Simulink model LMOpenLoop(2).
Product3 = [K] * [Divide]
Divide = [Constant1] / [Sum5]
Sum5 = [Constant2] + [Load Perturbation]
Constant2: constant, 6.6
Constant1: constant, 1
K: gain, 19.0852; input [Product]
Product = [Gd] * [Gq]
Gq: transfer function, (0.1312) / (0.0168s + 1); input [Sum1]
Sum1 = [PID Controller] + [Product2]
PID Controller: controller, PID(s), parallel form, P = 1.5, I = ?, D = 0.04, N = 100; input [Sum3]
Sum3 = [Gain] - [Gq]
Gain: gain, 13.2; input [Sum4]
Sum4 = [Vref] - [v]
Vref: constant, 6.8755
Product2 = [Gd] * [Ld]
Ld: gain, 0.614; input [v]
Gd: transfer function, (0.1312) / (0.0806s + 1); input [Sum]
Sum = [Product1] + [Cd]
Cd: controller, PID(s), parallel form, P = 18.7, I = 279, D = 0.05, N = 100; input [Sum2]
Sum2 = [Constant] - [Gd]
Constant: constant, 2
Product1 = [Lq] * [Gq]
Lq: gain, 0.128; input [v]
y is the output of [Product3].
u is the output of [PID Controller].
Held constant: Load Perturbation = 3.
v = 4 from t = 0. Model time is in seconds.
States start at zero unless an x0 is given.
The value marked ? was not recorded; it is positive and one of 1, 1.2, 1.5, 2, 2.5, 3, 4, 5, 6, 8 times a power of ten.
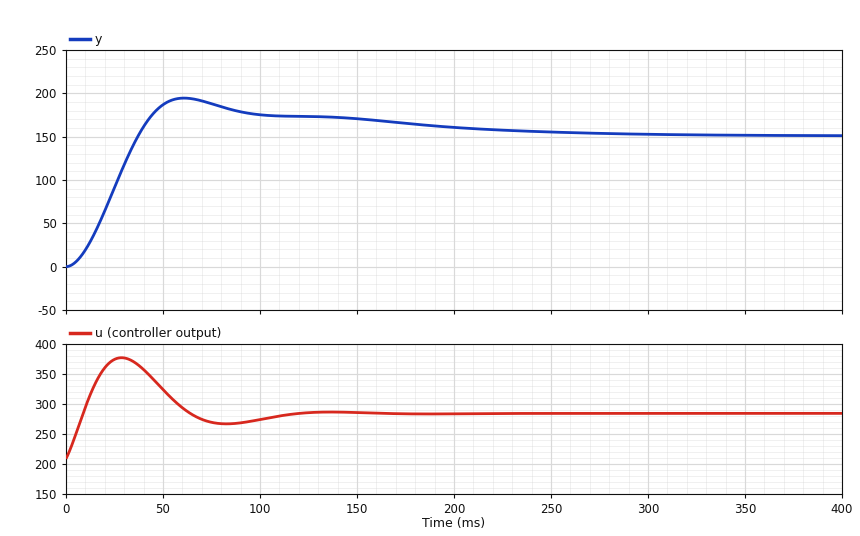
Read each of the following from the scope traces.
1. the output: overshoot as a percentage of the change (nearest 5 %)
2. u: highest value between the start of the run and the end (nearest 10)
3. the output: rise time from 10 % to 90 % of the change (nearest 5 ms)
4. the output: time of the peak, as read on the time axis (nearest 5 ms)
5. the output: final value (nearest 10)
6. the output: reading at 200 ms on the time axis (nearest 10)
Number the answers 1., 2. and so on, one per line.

1. 30 %
2. 380
3. 25 ms
4. 60 ms
5. 150
6. 160
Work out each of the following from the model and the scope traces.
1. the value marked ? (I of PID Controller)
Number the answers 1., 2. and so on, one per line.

1. 800
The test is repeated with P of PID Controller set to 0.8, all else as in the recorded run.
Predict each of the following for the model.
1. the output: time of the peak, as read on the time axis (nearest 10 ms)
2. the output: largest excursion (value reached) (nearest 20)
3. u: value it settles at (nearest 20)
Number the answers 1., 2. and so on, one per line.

1. 60 ms
2. 200
3. 280
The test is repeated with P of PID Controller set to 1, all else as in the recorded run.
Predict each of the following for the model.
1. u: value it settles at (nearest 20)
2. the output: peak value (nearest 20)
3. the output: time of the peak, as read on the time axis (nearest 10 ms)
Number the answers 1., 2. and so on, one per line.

1. 280
2. 200
3. 60 ms
